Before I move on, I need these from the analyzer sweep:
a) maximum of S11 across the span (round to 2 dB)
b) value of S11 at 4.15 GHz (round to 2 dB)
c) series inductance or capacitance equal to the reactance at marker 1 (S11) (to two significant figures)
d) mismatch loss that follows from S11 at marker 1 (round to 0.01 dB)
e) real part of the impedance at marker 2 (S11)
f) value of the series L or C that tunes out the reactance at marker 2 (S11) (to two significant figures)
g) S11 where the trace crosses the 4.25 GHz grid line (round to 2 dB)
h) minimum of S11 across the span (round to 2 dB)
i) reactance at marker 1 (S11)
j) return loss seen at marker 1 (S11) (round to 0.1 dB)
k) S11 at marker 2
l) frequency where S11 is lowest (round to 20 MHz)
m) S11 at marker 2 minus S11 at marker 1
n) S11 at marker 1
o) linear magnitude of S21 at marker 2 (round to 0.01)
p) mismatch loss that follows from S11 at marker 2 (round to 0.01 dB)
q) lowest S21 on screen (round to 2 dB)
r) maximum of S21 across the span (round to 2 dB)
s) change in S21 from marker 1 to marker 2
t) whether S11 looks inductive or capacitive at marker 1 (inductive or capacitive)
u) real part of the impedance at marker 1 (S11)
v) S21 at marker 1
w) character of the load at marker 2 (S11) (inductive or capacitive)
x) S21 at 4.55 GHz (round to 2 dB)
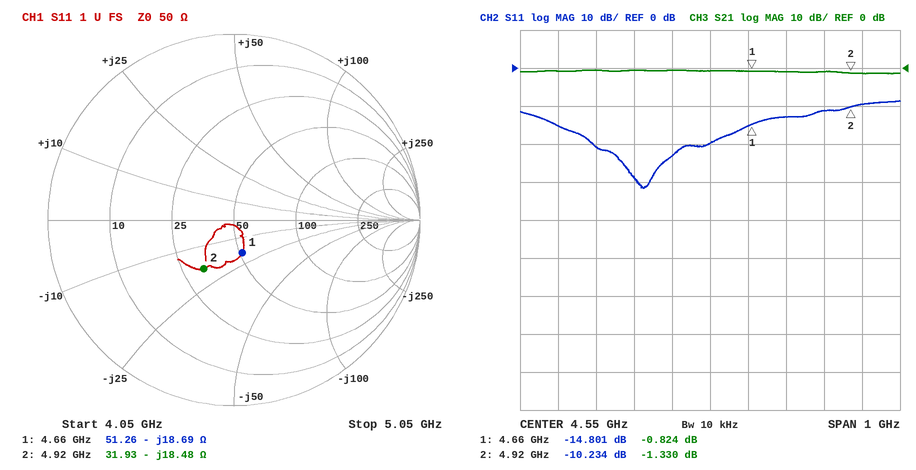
-8 dB
-16 dB
1.8 pF
0.15 dB
31.93 Ω
600 pH
-20 dB
-32 dB
-18.69 Ω
14.8 dB
-10.234 dB
4.38 GHz
4.567 dB
-14.801 dB
0.86
0.43 dB
-2 dB
0 dB
-0.506 dB
capacitive
51.26 Ω
-0.824 dB
capacitive
0 dB
